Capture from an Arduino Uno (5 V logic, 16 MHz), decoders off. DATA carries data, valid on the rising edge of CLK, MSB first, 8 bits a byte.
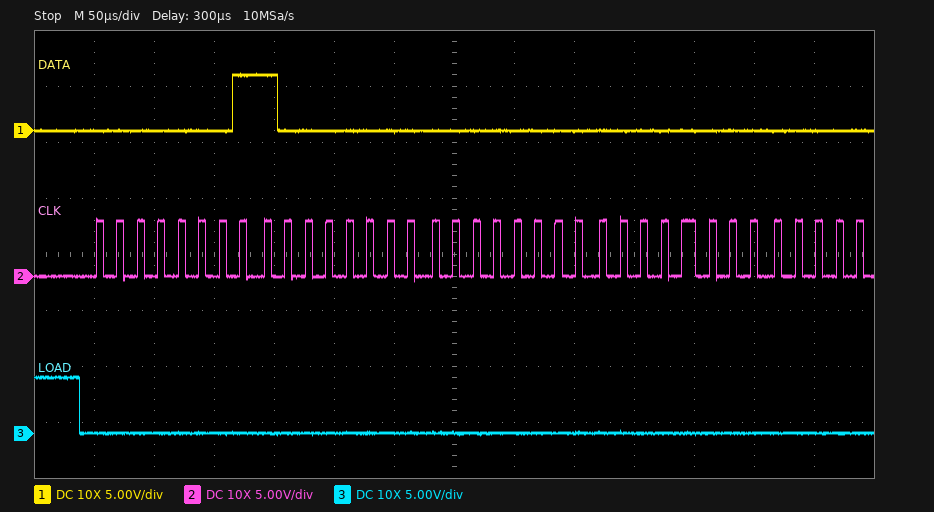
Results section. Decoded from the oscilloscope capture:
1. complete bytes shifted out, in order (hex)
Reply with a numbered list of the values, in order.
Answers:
1. 01 80 00 00
